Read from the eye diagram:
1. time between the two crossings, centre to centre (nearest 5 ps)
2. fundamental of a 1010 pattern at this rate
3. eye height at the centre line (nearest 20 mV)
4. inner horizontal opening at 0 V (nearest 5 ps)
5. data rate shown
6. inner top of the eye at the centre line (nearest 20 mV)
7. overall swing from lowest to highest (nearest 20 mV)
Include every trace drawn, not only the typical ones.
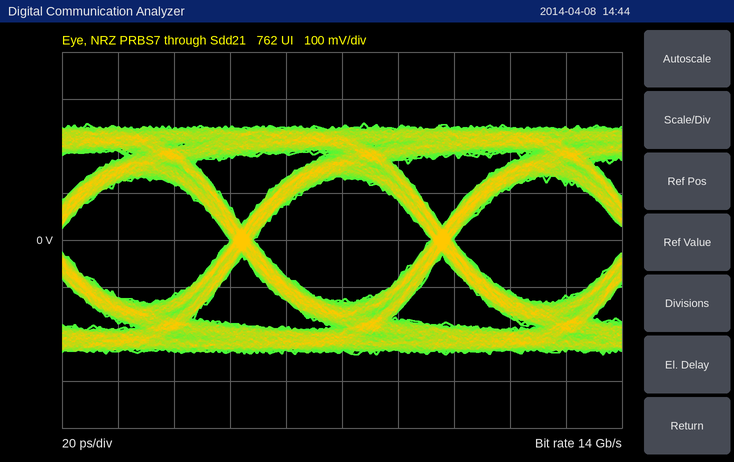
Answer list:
70 ps
7 GHz
260 mV
65 ps
14 Gb/s
140 mV
500 mV
